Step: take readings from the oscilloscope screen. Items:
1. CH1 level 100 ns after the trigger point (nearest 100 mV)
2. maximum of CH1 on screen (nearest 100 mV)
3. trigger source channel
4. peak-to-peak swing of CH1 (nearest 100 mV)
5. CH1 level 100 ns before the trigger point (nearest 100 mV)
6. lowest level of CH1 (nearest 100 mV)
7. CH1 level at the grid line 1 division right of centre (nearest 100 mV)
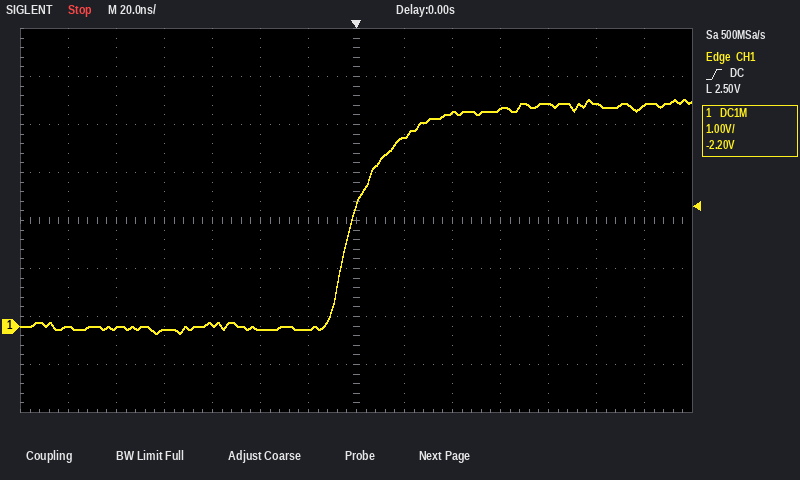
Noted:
4.6 V
4.7 V
CH1
4.9 V
0.0 V
-200 mV
3.9 V
